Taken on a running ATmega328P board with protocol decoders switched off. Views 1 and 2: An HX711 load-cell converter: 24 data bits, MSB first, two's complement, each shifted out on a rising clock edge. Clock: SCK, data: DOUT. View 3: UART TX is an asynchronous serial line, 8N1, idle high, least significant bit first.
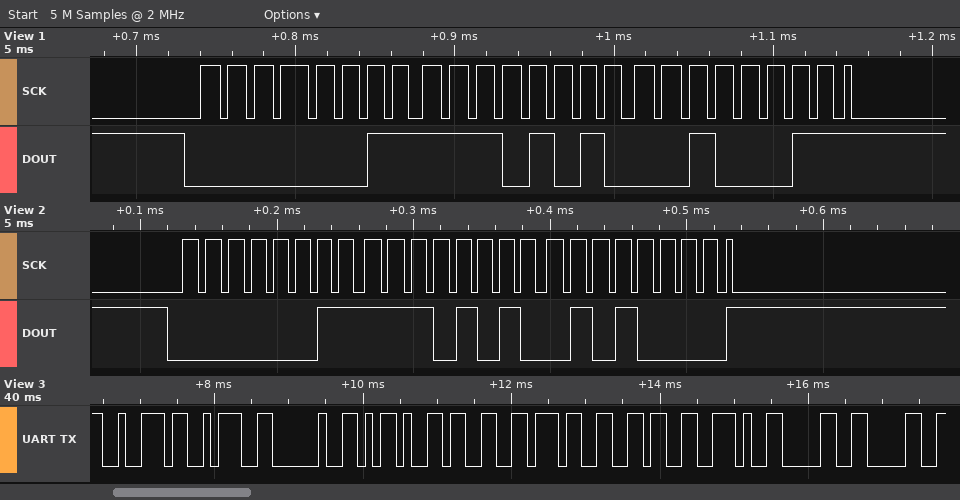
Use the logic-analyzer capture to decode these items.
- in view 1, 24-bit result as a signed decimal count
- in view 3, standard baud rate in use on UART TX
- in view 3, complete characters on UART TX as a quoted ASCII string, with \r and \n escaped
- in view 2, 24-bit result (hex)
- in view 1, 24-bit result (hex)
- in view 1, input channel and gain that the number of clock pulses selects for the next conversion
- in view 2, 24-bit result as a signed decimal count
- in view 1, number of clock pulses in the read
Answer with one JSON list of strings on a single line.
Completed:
["256547", "9600 baud", "\"r: -376.00\"", "0x03EA50", "0x03EA23", "channel A, gain 128", "256592", "25"]
